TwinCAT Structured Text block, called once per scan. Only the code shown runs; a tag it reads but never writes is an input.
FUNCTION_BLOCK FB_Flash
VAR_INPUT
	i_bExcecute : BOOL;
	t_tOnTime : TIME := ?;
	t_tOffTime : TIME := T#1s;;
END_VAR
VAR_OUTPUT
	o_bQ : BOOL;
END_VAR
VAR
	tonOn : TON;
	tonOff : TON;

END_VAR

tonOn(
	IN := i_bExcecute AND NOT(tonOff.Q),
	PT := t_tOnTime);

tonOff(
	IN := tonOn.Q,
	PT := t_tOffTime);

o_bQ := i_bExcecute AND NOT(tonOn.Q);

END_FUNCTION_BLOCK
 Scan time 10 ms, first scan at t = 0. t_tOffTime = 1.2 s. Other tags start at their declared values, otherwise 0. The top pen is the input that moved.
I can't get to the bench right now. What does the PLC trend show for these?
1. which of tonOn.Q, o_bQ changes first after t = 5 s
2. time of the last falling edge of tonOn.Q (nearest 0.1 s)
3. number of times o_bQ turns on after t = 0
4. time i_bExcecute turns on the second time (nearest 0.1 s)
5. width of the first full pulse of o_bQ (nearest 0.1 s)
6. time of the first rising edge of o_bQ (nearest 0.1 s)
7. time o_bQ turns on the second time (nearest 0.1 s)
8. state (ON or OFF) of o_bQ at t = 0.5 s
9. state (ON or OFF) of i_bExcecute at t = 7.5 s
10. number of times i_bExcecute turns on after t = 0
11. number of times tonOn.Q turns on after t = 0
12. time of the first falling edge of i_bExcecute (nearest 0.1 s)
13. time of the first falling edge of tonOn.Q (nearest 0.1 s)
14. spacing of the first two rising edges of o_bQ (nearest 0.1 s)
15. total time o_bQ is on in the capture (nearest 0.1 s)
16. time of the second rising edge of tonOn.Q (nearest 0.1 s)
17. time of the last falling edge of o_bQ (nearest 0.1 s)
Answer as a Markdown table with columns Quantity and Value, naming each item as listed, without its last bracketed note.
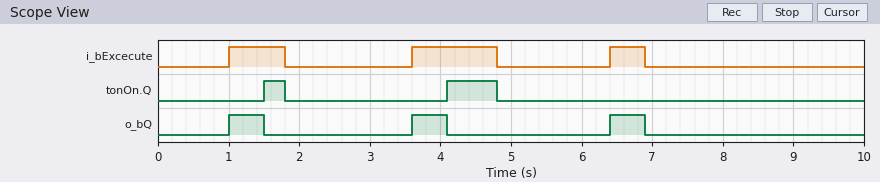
| Quantity | Value |
|---|---|
| which of tonOn.Q, o_bQ changes first after t = 5 s | o_bQ |
| time of the last falling edge of tonOn.Q | 4.8 s |
| number of times o_bQ turns on after t = 0 | 3 |
| time i_bExcecute turns on the second time | 3.6 s |
| width of the first full pulse of o_bQ | 0.5 s |
| time of the first rising edge of o_bQ | 1.0 s |
| time o_bQ turns on the second time | 3.6 s |
| state (ON or OFF) of o_bQ at t = 0.5 s | OFF |
| state (ON or OFF) of i_bExcecute at t = 7.5 s | OFF |
| number of times i_bExcecute turns on after t = 0 | 3 |
| number of times tonOn.Q turns on after t = 0 | 2 |
| time of the first falling edge of i_bExcecute | 1.8 s |
| time of the first falling edge of tonOn.Q | 1.8 s |
| spacing of the first two rising edges of o_bQ | 2.6 s |
| total time o_bQ is on in the capture | 1.5 s |
| time of the second rising edge of tonOn.Q | 4.1 s |
| time of the last falling edge of o_bQ | 6.9 s |
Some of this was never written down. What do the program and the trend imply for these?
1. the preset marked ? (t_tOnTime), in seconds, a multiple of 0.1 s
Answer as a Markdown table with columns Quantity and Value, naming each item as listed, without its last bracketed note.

| Quantity | Value |
|---|---|
| the preset marked ? (t_tOnTime), in seconds, a multiple of 0.1 s | 0.5 s |
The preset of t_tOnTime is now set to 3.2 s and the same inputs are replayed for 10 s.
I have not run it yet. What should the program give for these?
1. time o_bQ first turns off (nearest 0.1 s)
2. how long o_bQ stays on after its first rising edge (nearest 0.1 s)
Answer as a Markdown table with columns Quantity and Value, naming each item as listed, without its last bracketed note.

| Quantity | Value |
|---|---|
| time o_bQ first turns off | 1.8 s |
| how long o_bQ stays on after its first rising edge | 0.8 s |
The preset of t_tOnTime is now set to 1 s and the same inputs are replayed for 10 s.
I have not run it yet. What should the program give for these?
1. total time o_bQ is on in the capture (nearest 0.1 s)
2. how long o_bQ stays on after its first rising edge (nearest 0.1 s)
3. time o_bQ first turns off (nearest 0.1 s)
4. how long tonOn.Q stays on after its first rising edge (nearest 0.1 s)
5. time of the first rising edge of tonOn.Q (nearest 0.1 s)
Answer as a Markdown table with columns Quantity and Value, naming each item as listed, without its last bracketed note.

| Quantity | Value |
|---|---|
| total time o_bQ is on in the capture | 2.3 s |
| how long o_bQ stays on after its first rising edge | 0.8 s |
| time o_bQ first turns off | 1.8 s |
| how long tonOn.Q stays on after its first rising edge | 0.2 s |
| time of the first rising edge of tonOn.Q | 4.6 s |
